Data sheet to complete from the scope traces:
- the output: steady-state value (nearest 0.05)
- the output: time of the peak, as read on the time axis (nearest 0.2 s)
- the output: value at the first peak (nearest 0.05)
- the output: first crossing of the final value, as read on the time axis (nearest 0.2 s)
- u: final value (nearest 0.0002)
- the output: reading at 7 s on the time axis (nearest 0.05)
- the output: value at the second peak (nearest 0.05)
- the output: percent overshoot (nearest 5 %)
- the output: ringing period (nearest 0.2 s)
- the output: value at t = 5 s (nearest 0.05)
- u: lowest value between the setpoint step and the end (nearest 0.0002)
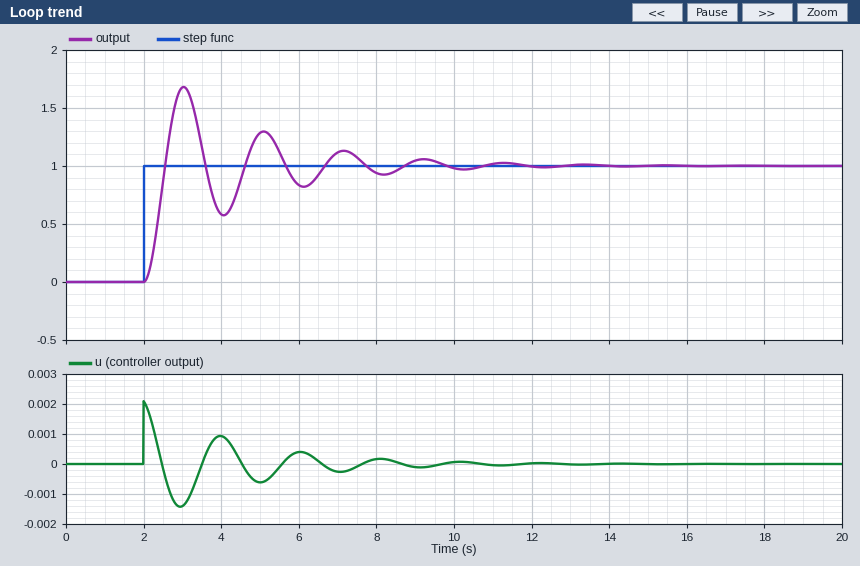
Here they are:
1.00
3.0 s
1.70
2.6 s
0.0000
1.10
1.30
70 %
2.0 s
1.30
-0.0014
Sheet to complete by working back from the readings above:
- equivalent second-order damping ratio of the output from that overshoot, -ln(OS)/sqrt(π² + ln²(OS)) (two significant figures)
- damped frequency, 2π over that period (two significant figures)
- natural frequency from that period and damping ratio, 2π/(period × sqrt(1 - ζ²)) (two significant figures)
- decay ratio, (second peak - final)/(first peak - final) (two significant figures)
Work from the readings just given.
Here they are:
0.11
3.1 rad/s
3.2 rad/s
0.43
